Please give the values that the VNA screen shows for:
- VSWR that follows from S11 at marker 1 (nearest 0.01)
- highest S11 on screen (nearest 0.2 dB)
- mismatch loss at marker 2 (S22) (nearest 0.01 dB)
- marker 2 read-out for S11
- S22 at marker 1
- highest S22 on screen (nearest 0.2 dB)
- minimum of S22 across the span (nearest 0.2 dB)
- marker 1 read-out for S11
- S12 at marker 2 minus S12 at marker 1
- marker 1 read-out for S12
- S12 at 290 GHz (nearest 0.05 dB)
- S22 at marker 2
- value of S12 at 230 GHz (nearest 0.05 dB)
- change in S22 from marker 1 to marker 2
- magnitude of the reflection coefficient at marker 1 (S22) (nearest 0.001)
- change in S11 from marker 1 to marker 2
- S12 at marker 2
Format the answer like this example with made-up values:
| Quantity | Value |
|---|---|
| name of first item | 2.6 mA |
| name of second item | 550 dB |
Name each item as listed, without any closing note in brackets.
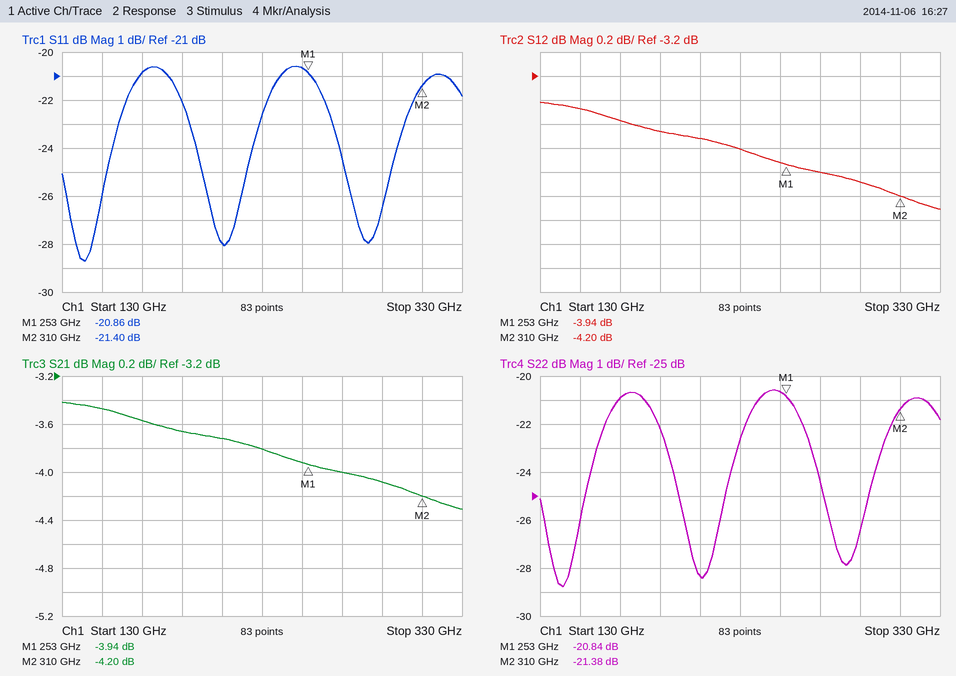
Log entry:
| Quantity | Value |
|---|---|
| VSWR that follows from S11 at marker 1 | 1.20 |
| highest S11 on screen | -20.6 dB |
| mismatch loss at marker 2 (S22) | 0.03 dB |
| marker 2 read-out for S11 | -21.40 dB |
| S22 at marker 1 | -20.84 dB |
| highest S22 on screen | -20.6 dB |
| minimum of S22 across the span | -28.8 dB |
| marker 1 read-out for S11 | -20.86 dB |
| S12 at marker 2 minus S12 at marker 1 | -0.26 dB |
| marker 1 read-out for S12 | -3.94 dB |
| S12 at 290 GHz | -4.10 dB |
| S22 at marker 2 | -21.38 dB |
| value of S12 at 230 GHz | -3.80 dB |
| change in S22 from marker 1 to marker 2 | -0.54 dB |
| magnitude of the reflection coefficient at marker 1 (S22) | 0.091 |
| change in S11 from marker 1 to marker 2 | -0.54 dB |
| S12 at marker 2 | -4.20 dB |
